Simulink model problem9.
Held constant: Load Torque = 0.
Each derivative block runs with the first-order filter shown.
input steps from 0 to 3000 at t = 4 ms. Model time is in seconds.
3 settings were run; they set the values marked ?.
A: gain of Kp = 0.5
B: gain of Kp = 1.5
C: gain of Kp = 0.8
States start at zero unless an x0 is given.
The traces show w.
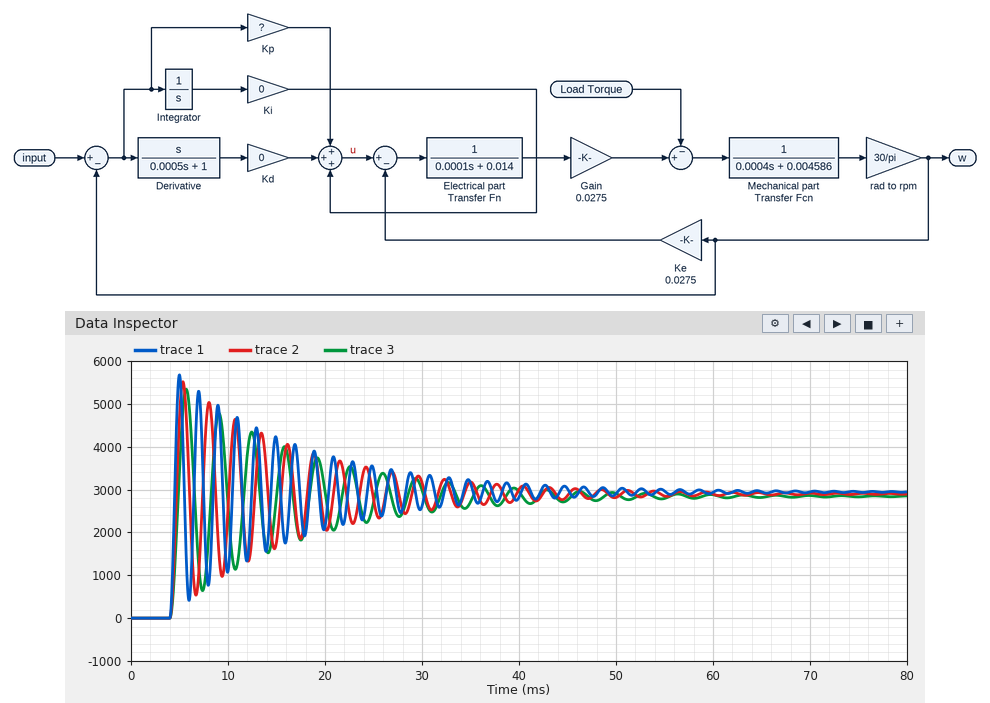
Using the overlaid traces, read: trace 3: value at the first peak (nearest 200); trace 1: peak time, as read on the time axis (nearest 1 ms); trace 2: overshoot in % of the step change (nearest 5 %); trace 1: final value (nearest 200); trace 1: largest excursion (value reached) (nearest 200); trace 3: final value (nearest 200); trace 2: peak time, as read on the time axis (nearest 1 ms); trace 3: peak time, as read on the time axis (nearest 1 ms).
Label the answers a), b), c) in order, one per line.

a) 5400
b) 5 ms
c) 90 %
d) 3000
e) 5600
f) 2800
g) 5 ms
h) 6 ms
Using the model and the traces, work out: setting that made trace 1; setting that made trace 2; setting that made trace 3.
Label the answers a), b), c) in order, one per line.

a) B
b) C
c) A
